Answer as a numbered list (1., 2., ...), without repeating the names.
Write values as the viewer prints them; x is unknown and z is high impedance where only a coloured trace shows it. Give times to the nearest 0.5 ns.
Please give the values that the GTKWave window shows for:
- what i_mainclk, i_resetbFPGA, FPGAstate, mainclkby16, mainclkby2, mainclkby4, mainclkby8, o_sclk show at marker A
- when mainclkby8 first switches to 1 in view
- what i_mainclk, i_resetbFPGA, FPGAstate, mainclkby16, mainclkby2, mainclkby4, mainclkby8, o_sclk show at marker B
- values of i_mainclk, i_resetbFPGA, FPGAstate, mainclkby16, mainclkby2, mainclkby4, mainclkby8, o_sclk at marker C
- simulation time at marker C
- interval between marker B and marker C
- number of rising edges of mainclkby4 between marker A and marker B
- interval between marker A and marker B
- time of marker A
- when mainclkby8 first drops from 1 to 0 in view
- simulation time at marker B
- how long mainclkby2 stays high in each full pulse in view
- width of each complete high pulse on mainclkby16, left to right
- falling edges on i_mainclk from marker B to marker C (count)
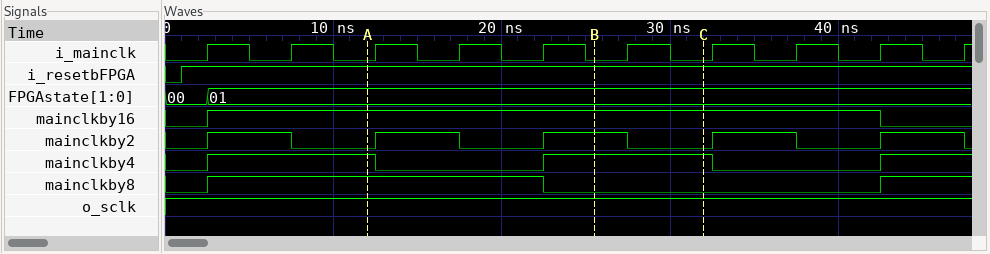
1. i_mainclk=0, i_resetbFPGA=1, FPGAstate=01, mainclkby16=1, mainclkby2=0, mainclkby4=1, mainclkby8=1, o_sclk=1
2. 2.5 ns
3. i_mainclk=0, i_resetbFPGA=1, FPGAstate=01, mainclkby16=1, mainclkby2=1, mainclkby4=1, mainclkby8=0, o_sclk=1
4. i_mainclk=0, i_resetbFPGA=1, FPGAstate=01, mainclkby16=1, mainclkby2=0, mainclkby4=1, mainclkby8=0, o_sclk=1
5. 32 ns
6. 6.5 ns
7. 1
8. 13.5 ns
9. 12 ns
10. 22.5 ns
11. 25.5 ns
12. 5 ns, 5 ns, 5 ns, 5 ns, 5 ns
13. 40 ns
14. 1
